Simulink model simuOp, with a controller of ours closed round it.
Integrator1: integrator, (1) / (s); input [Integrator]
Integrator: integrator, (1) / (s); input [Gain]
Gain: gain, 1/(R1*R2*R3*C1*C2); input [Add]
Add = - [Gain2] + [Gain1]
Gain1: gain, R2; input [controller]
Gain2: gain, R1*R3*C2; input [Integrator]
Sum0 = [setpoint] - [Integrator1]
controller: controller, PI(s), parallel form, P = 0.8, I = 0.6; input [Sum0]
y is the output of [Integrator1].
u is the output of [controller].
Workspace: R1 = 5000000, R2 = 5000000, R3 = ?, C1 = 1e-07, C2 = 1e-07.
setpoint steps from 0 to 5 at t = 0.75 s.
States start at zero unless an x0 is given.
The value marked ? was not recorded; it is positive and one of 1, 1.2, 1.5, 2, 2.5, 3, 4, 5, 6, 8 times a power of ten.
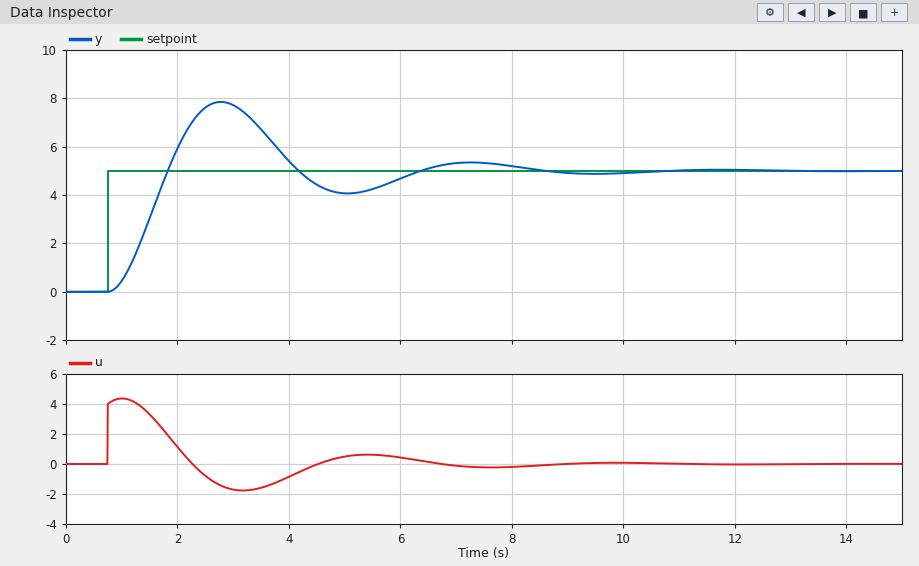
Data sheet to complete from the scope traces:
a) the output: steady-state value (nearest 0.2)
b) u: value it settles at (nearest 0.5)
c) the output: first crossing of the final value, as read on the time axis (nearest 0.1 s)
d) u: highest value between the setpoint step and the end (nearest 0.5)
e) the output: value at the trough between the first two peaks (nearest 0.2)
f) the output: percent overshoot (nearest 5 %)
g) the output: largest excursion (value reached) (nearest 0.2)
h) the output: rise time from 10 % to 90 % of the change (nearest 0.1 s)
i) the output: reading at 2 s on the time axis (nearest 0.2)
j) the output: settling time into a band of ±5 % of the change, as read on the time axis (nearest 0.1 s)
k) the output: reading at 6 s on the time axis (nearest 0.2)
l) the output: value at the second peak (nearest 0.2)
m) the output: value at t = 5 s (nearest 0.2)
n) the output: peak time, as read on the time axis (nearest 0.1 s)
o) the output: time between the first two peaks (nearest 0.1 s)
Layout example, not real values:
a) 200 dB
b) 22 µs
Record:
a) 5.0
b) 0.0
c) 1.8 s
d) 4.5
e) 4.0
f) 55 %
g) 7.8
h) 0.7 s
i) 6.0
j) 7.8 s
k) 4.6
l) 5.4
m) 4.0
n) 2.8 s
o) 4.5 s
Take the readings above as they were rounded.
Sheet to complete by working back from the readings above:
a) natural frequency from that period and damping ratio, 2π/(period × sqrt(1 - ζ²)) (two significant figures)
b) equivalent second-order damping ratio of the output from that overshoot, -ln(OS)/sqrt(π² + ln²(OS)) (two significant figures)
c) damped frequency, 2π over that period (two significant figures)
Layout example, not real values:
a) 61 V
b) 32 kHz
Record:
a) 1.4 rad/s
b) 0.19
c) 1.4 rad/s
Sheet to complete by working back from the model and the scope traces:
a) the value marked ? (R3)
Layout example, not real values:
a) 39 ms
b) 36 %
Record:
a) 5e+06
